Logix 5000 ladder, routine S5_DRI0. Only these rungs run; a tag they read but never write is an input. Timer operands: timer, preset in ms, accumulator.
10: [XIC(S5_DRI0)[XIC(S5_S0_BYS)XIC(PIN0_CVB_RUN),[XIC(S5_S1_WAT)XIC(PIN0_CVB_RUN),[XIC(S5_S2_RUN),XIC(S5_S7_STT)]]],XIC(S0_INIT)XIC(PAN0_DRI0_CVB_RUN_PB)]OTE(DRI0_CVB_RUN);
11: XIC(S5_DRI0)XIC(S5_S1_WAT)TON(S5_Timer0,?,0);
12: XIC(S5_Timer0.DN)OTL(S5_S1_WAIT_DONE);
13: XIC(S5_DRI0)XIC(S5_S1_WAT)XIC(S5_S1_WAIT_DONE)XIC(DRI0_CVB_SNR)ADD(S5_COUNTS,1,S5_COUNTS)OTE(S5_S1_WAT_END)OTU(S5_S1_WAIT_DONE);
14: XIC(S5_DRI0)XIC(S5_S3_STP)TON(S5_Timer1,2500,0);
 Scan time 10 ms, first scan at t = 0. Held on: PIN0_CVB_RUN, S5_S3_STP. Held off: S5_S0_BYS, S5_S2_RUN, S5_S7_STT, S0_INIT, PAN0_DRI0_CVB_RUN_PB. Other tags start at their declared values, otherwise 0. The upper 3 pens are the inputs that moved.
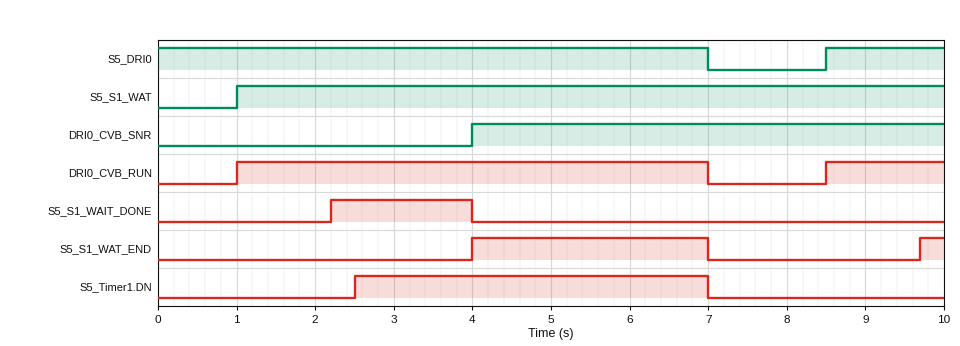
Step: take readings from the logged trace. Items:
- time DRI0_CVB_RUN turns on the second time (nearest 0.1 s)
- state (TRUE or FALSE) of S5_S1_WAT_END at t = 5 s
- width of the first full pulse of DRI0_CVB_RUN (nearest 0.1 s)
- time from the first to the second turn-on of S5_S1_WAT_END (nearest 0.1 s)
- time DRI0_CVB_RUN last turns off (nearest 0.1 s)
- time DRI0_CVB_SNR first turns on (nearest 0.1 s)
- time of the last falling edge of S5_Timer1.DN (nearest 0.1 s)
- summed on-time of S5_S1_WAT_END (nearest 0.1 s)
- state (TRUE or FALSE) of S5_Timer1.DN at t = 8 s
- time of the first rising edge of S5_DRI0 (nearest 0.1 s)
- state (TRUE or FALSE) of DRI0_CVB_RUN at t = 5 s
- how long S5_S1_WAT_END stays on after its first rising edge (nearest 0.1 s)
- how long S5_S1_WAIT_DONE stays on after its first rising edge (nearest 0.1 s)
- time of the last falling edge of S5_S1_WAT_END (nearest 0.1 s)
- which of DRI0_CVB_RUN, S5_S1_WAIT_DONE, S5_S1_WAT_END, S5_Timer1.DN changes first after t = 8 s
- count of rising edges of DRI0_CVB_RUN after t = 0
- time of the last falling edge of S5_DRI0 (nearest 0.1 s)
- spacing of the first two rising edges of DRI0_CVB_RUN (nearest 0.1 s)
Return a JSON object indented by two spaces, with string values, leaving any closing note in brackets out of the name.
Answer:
{
  "time DRI0_CVB_RUN turns on the second time": "8.5 s",
  "state (TRUE or FALSE) of S5_S1_WAT_END at t = 5 s": "TRUE",
  "width of the first full pulse of DRI0_CVB_RUN": "6.0 s",
  "time from the first to the second turn-on of S5_S1_WAT_END": "5.7 s",
  "time DRI0_CVB_RUN last turns off": "7.0 s",
  "time DRI0_CVB_SNR first turns on": "4.0 s",
  "time of the last falling edge of S5_Timer1.DN": "7.0 s",
  "summed on-time of S5_S1_WAT_END": "3.3 s",
  "state (TRUE or FALSE) of S5_Timer1.DN at t = 8 s": "FALSE",
  "time of the first rising edge of S5_DRI0": "8.5 s",
  "state (TRUE or FALSE) of DRI0_CVB_RUN at t = 5 s": "TRUE",
  "how long S5_S1_WAT_END stays on after its first rising edge": "3.0 s",
  "how long S5_S1_WAIT_DONE stays on after its first rising edge": "1.8 s",
  "time of the last falling edge of S5_S1_WAT_END": "7.0 s",
  "which of DRI0_CVB_RUN, S5_S1_WAIT_DONE, S5_S1_WAT_END, S5_Timer1.DN changes first after t = 8 s": "DRI0_CVB_RUN",
  "count of rising edges of DRI0_CVB_RUN after t = 0": "2",
  "time of the last falling edge of S5_DRI0": "7.0 s",
  "spacing of the first two rising edges of DRI0_CVB_RUN": "7.5 s"
}
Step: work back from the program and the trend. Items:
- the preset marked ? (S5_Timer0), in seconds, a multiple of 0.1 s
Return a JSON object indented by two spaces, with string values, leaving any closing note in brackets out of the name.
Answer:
{
  "the preset marked ? (S5_Timer0), in seconds, a multiple of 0.1 s": "1.2 s"
}
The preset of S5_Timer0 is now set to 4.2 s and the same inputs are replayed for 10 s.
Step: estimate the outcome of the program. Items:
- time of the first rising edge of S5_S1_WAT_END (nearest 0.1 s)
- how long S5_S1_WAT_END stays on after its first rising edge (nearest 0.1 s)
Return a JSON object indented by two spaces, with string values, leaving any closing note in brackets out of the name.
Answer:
{
  "time of the first rising edge of S5_S1_WAT_END": "5.2 s",
  "how long S5_S1_WAT_END stays on after its first rising edge": "1.8 s"
}
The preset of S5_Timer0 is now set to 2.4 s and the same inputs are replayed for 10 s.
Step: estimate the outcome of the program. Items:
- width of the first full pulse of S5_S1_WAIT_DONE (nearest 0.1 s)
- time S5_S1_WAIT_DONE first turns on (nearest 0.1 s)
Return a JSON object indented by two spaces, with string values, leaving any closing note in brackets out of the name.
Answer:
{
  "width of the first full pulse of S5_S1_WAIT_DONE": "0.6 s",
  "time S5_S1_WAIT_DONE first turns on": "3.4 s"
}
